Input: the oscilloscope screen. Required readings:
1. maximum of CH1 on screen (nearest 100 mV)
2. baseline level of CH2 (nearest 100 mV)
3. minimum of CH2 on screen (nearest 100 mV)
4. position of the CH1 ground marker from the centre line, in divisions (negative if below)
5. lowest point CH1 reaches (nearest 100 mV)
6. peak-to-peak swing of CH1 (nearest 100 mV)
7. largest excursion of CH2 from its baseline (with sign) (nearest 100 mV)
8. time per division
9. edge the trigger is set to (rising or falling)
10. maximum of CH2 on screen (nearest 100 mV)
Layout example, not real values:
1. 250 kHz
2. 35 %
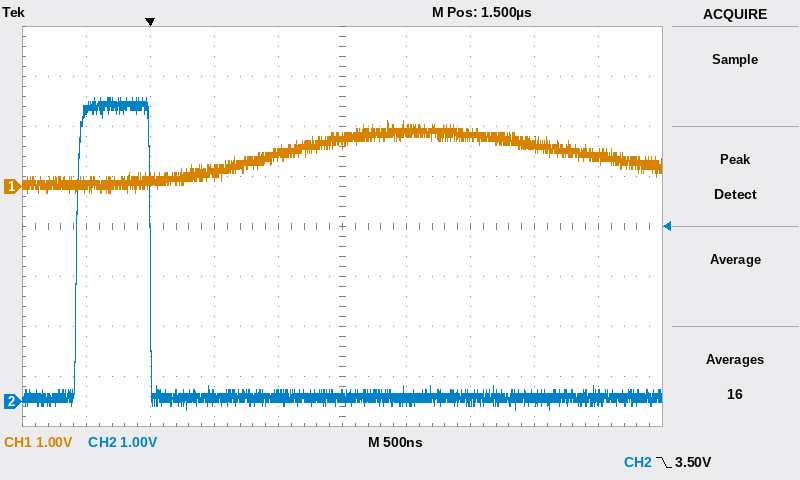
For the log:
1. 1.3 V
2. 100 mV
3. -200 mV
4. +0.8 div
5. -100 mV
6. 1.4 V
7. +6.0 V
8. 500 ns
9. falling
10. 6.1 V
